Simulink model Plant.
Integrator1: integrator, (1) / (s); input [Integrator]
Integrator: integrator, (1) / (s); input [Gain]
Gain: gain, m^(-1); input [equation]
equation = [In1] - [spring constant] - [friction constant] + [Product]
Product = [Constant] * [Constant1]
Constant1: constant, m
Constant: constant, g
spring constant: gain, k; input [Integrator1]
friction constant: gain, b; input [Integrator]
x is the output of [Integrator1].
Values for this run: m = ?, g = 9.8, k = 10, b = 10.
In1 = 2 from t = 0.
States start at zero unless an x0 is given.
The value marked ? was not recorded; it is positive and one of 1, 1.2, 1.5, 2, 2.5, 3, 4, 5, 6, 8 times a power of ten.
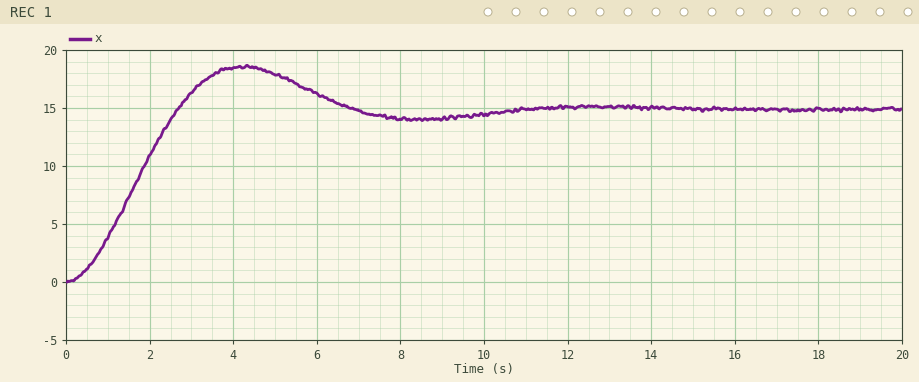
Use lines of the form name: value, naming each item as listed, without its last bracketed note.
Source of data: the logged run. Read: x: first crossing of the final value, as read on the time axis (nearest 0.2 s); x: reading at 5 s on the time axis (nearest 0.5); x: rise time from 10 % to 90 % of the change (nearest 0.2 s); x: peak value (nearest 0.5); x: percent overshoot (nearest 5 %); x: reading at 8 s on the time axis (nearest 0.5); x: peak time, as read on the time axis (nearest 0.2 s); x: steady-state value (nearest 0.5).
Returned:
x: first crossing of the final value, as read on the time axis: 2.6 s
x: reading at 5 s on the time axis: 18.0
x: rise time from 10 % to 90 % of the change: 1.8 s
x: peak value: 18.5
x: percent overshoot: 25 %
x: reading at 8 s on the time axis: 14.0
x: peak time, as read on the time axis: 4.2 s
x: steady-state value: 15.0
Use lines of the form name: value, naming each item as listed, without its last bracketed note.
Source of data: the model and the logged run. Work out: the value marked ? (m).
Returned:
the value marked ?: 15
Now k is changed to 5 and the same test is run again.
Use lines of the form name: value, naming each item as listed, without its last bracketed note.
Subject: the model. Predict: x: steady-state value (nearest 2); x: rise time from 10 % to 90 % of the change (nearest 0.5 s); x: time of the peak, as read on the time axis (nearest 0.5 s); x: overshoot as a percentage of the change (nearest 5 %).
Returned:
x: steady-state value: 30
x: rise time from 10 % to 90 % of the change: 3.0 s
x: time of the peak, as read on the time axis: 6.5 s
x: overshoot as a percentage of the change: 10 %
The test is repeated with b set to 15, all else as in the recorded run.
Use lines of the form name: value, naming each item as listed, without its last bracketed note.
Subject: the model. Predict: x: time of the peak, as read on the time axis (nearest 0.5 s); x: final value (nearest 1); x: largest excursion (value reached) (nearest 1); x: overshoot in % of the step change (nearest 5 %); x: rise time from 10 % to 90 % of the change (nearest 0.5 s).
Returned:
x: time of the peak, as read on the time axis: 5.0 s
x: final value: 15
x: largest excursion (value reached): 16
x: overshoot in % of the step change: 10 %
x: rise time from 10 % to 90 % of the change: 2.5 s
